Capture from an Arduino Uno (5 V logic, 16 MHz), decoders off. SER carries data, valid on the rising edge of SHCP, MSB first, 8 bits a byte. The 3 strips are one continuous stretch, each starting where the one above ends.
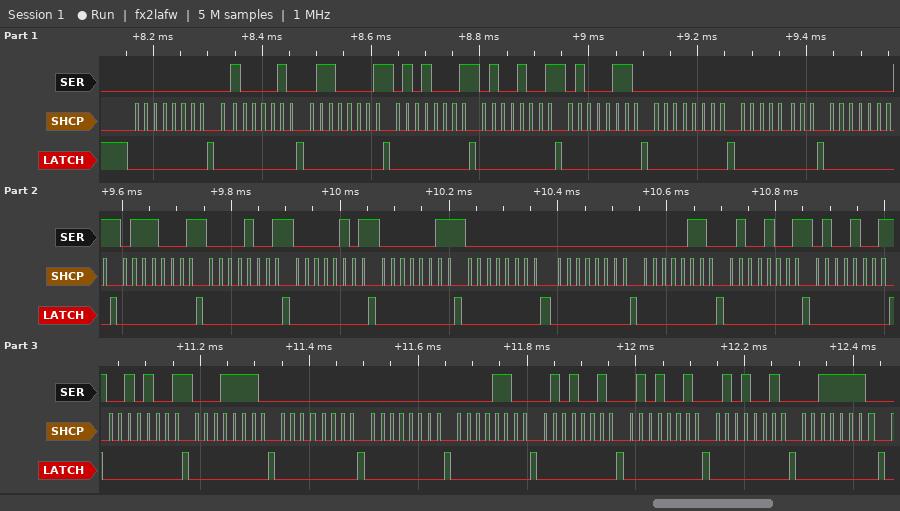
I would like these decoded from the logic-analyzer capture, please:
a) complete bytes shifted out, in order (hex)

0x00 0x42 0x61 0x51 0x49 0x46 0x00 0x00 0x01 0x71 0x09 0x05 0x03 0x00 0x00 0x06 0x49 0x49 0x29 0x1E 0x00 0x00 0x0C 0x52 0x52 0x52 0x3E
